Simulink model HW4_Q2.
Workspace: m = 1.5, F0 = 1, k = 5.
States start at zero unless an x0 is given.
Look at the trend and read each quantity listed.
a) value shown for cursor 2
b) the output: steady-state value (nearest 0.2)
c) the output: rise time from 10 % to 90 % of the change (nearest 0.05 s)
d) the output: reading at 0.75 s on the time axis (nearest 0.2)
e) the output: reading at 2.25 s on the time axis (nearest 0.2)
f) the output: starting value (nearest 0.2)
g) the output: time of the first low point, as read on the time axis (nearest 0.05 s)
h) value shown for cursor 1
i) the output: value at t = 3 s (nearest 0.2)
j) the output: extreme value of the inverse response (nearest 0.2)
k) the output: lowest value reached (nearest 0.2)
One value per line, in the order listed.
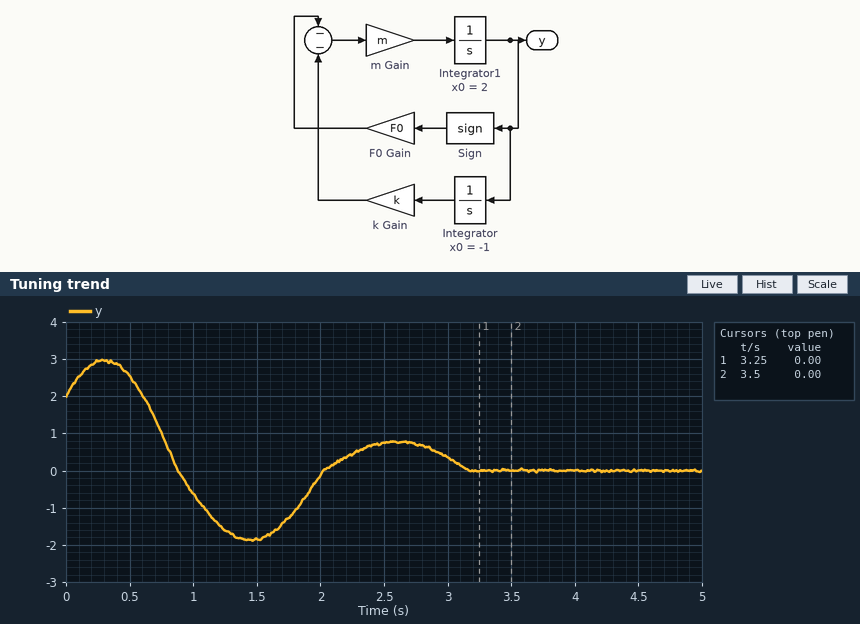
0.00
0.0
0.20 s
1.0
0.4
2.0
1.45 s
0.00
0.4
3.0
-1.8
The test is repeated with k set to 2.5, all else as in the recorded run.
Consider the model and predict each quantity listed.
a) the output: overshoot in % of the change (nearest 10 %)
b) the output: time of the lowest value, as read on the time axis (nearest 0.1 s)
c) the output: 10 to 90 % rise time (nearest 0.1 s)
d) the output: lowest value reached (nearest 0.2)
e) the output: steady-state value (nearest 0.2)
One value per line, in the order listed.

40 %
1.9 s
0.4 s
-0.8
0.0
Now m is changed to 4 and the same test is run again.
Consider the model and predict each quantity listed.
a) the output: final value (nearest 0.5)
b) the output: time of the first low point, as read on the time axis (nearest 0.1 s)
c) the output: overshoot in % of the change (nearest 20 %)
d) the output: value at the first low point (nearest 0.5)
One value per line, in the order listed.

0.0
0.9 s
120 %
-2.5
